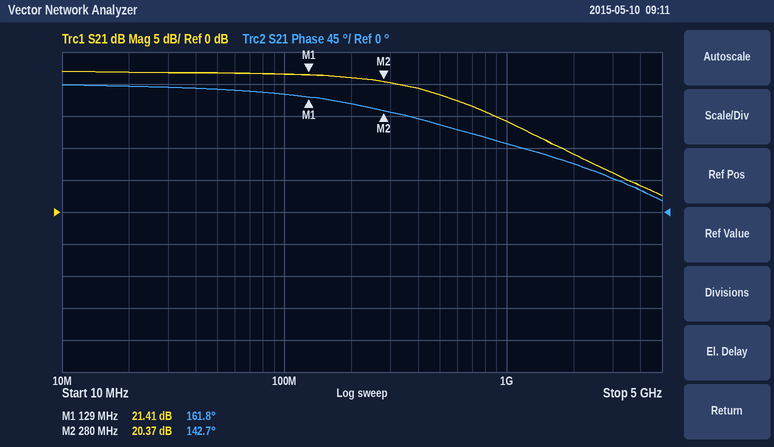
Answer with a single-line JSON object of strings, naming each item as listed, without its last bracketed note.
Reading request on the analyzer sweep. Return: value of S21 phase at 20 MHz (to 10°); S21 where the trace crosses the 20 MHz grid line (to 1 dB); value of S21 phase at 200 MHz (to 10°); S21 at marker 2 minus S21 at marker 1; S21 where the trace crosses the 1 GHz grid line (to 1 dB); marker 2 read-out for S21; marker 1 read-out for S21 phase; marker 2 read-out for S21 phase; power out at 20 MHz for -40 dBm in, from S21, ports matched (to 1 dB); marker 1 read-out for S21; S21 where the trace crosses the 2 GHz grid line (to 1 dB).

{"value of S21 phase at 20 MHz": "180°", "S21 where the trace crosses the 20 MHz grid line": "22 dB", "value of S21 phase at 200 MHz": "150°", "S21 at marker 2 minus S21 at marker 1": "-1.04 dB", "S21 where the trace crosses the 1 GHz grid line": "14 dB", "marker 2 read-out for S21": "20.37 dB", "marker 1 read-out for S21 phase": "161.8°", "marker 2 read-out for S21 phase": "142.7°", "power out at 20 MHz for -40 dBm in, from S21, ports matched": "-18 dBm", "marker 1 read-out for S21": "21.41 dB", "S21 where the trace crosses the 2 GHz grid line": "9 dB"}
